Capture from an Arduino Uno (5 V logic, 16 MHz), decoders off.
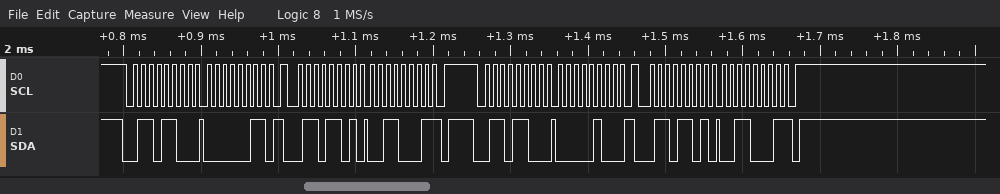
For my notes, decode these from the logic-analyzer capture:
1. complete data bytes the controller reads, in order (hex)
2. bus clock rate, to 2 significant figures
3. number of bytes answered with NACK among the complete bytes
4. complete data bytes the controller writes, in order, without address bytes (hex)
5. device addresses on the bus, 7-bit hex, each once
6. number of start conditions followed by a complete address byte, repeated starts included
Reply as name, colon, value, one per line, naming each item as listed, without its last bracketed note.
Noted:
complete data bytes the controller reads, in order: 31 31
bus clock rate, to 2 significant figures: 100 kHz
number of bytes answered with NACK among the complete bytes: 2
complete data bytes the controller writes, in order, without address bytes: 03 04
device addresses on the bus, 7-bit hex, each once: 0x36
number of start conditions followed by a complete address byte, repeated starts included: 4
